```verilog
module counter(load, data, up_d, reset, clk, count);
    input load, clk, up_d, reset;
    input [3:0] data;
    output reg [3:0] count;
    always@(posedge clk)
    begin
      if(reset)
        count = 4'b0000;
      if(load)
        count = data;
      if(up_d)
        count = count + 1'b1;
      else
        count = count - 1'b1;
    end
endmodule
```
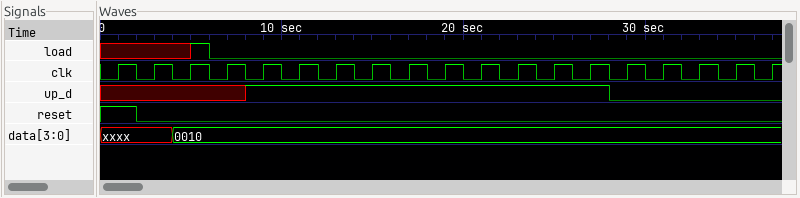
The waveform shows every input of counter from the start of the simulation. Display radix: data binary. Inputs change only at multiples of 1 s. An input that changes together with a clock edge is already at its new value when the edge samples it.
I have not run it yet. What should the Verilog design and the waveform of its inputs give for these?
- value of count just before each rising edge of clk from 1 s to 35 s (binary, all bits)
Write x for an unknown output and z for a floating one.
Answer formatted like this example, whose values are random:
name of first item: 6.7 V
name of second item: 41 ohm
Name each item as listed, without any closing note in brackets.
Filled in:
value of count just before each rising edge of clk from 1 s to 35 s: x, 1111, 1110, 0001, 0000, 0001, 0010, 0011, 0100, 0101, 0110, 0111, 1000, 1001, 1010, 1001, 1000, 0111
